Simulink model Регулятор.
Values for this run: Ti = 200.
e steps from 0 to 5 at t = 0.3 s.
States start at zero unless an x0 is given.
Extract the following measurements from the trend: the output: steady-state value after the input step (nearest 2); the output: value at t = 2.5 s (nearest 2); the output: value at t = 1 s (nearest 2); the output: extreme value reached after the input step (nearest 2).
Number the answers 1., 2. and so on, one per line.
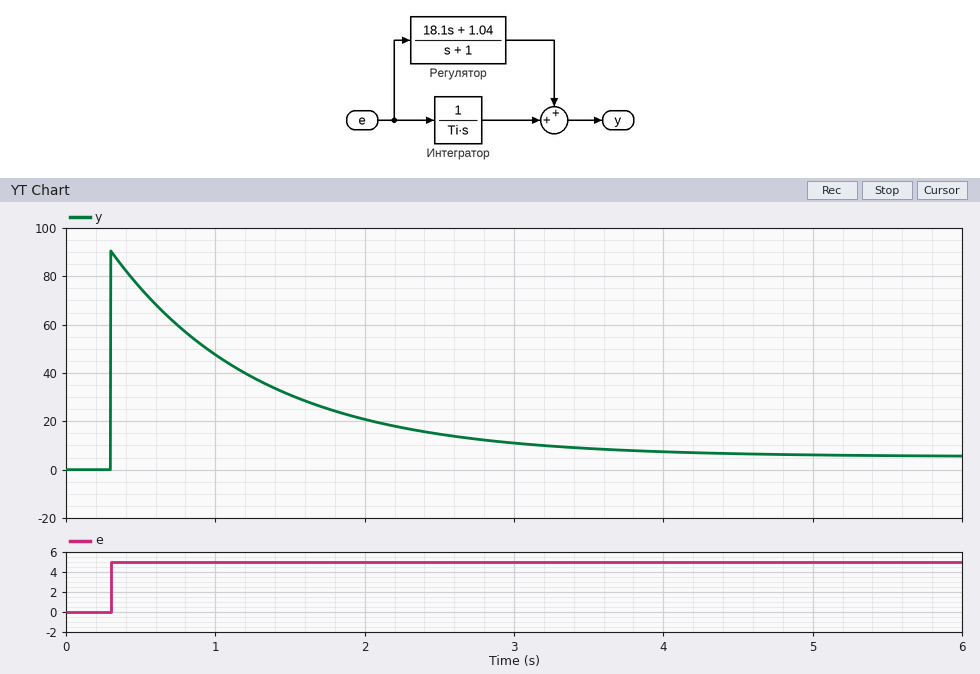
1. 6
2. 14
3. 48
4. 90
